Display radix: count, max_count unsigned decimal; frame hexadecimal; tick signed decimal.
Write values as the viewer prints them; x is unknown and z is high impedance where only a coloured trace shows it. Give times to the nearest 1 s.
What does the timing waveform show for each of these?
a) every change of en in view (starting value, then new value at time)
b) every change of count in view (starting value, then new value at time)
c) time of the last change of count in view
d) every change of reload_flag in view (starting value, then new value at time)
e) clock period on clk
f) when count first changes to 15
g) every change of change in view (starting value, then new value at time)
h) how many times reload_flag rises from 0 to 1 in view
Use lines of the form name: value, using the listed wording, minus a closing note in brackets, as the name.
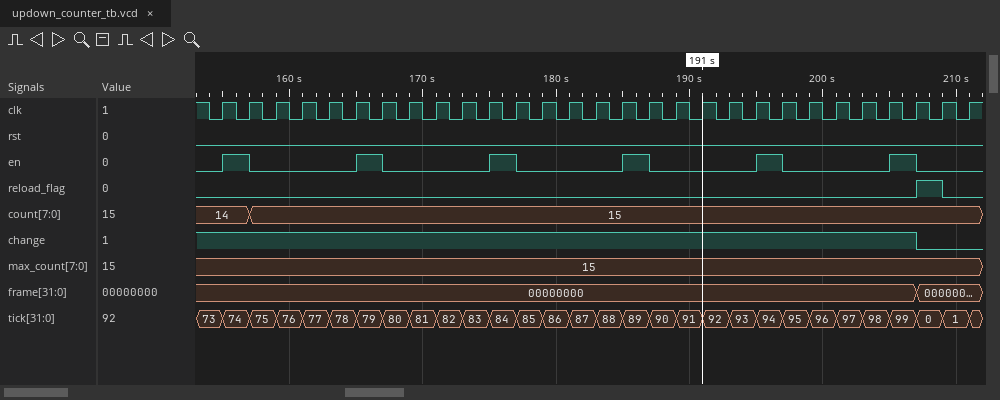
every change of en in view: 0, 1 at 155 s, 0 at 157 s, 1 at 165 s, 0 at 167 s, 1 at 175 s, 0 at 177 s, 1 at 185 s, 0 at 187 s, 1 at 195 s, 0 at 197 s, 1 at 205 s, 0 at 207 s
every change of count in view: 14, 15 at 157 s
time of the last change of count in view: 157 s
every change of reload_flag in view: 0, 1 at 207 s, 0 at 209 s
clock period on clk: 2 s
when count first changes to 15: 157 s
every change of change in view: 1, 0 at 207 s
how many times reload_flag rises from 0 to 1 in view: 1
